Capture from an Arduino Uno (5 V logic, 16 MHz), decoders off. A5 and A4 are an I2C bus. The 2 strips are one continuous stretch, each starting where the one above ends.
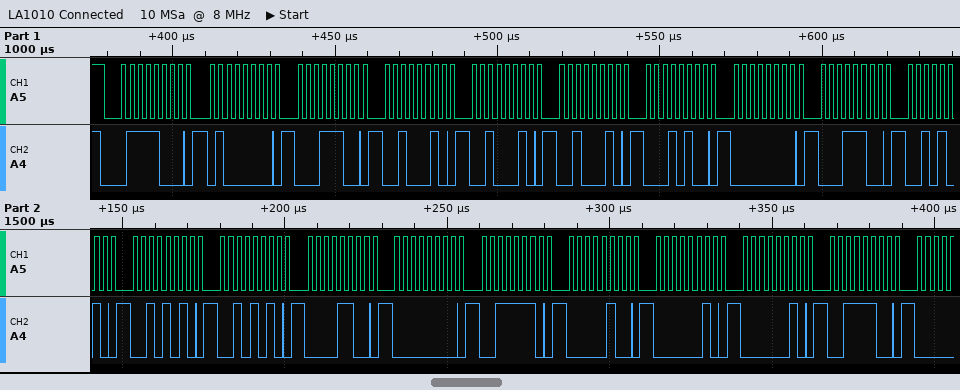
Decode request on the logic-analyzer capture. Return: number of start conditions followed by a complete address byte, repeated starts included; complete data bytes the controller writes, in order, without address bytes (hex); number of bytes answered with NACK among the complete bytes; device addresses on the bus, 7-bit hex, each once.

1
40 1C 22 22 22 14 00 1C 2A 2A 2A 0C 00 3E 04 02 02 3C
0
0x3C
